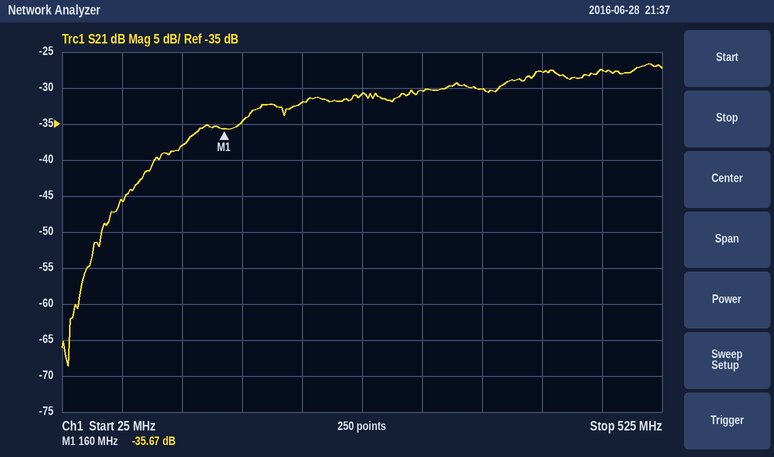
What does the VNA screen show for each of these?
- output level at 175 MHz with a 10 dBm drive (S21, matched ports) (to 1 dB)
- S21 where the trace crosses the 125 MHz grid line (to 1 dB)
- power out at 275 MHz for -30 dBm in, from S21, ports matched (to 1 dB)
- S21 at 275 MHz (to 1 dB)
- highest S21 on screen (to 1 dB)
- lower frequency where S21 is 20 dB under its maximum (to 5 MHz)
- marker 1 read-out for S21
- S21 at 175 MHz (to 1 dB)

-25 dBm
-38 dB
-61 dBm
-31 dB
-27 dB
70 MHz
-35.67 dB
-35 dB
